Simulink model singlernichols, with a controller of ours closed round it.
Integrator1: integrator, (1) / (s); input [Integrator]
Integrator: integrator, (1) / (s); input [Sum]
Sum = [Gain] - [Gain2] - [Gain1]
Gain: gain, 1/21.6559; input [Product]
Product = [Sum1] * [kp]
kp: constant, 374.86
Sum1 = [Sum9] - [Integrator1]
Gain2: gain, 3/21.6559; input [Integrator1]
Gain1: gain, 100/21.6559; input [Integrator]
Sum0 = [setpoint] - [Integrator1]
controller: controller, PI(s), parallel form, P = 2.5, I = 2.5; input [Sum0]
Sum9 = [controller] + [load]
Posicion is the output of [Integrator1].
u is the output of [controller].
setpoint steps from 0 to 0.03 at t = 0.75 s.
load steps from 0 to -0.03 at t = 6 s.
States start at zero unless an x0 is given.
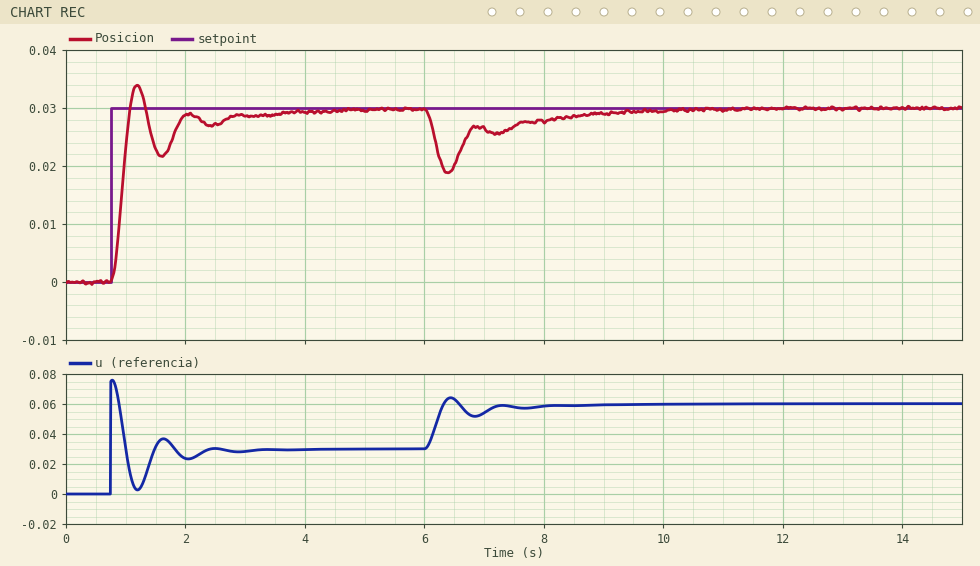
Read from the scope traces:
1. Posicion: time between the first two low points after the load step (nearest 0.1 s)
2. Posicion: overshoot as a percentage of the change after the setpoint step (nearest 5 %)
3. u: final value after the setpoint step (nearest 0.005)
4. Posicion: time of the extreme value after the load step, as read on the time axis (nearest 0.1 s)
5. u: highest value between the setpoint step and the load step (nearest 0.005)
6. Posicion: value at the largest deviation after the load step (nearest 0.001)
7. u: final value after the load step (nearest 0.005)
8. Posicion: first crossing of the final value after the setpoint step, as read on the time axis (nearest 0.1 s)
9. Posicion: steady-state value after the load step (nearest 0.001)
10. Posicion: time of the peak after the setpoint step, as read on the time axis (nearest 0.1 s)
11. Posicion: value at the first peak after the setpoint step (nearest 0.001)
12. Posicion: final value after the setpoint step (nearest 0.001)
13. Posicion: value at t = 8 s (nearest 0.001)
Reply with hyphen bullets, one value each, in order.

- 0.8 s
- 15 %
- 0.030
- 6.4 s
- 0.075
- 0.019
- 0.060
- 1.1 s
- 0.030
- 1.2 s
- 0.034
- 0.030
- 0.028
